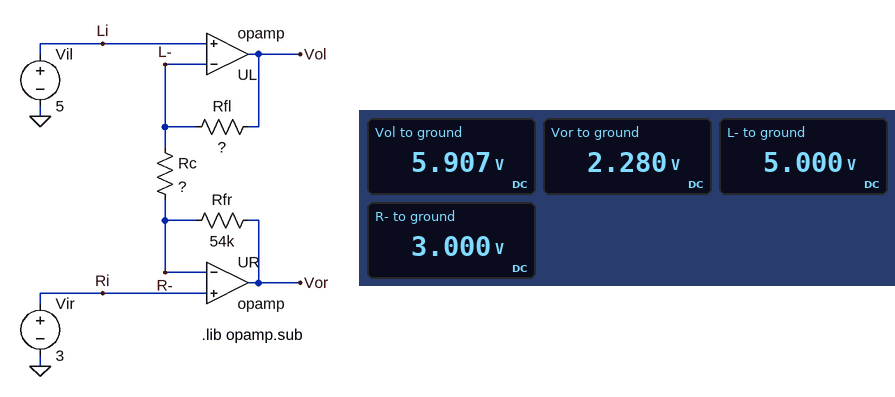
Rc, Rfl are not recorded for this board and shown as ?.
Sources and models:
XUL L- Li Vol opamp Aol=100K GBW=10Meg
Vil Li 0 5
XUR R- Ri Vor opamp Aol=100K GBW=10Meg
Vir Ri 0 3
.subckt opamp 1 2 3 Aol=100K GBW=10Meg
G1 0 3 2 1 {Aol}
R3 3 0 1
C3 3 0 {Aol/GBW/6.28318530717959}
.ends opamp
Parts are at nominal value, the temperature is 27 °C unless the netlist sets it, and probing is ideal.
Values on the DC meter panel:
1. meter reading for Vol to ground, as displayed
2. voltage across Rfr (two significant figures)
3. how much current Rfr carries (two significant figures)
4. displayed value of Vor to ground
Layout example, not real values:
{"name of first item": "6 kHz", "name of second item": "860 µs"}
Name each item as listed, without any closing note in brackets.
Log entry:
{"meter reading for Vol to ground, as displayed": "5.907 V", "voltage across Rfr": "720 mV", "how much current Rfr carries": "13 µA", "displayed value of Vor to ground": "2.280 V"}
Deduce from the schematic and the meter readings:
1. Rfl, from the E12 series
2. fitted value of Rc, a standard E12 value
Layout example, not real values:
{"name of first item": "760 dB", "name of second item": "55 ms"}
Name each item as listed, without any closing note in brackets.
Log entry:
{"Rfl, from the E12 series": "68 kΩ", "fitted value of Rc, a standard E12 value": "150 kΩ"}
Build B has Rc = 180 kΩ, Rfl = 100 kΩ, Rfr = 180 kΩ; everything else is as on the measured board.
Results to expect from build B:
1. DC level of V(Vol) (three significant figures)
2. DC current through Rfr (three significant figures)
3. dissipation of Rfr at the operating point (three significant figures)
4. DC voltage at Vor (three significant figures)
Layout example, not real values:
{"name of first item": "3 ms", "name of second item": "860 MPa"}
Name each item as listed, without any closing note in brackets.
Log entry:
{"DC level of V(Vol)": "6.11 V", "DC current through Rfr": "11.1 µA", "dissipation of Rfr at the operating point": "22.2 µW", "DC voltage at Vor": "1.00 V"}
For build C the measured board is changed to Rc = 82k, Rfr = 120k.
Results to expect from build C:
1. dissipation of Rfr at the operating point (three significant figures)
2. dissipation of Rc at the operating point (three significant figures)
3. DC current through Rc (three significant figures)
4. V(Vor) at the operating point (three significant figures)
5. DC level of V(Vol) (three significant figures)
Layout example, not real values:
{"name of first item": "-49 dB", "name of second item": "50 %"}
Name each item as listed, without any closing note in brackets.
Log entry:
{"dissipation of Rfr at the operating point": "71.4 µW", "dissipation of Rc at the operating point": "48.8 µW", "DC current through Rc": "24.4 µA", "V(Vor) at the operating point": "73.3 mV", "DC level of V(Vol)": "6.66 V"}
